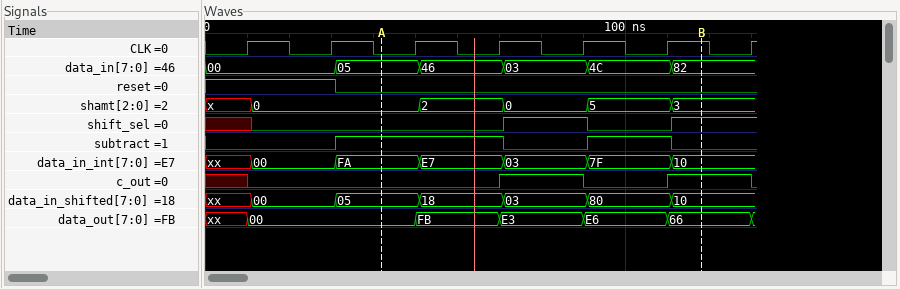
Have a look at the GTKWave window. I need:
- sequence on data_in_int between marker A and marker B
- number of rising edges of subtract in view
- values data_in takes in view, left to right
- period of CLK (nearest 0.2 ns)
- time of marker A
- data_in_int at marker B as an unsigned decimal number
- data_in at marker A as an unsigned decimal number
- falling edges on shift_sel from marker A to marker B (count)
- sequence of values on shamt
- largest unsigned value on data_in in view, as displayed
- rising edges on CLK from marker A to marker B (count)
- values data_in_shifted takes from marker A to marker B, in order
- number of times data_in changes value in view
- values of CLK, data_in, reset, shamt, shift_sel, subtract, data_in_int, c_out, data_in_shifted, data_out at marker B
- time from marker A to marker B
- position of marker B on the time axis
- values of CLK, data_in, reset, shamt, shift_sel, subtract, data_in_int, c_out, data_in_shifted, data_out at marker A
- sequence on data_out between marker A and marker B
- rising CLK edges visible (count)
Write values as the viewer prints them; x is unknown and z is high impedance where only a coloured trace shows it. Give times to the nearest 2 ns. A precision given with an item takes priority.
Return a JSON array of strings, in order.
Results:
["FA, E7, 03, 7F, 10", "2", "00, 05, 46, 03, 4C, 82", "20 ns", "42 ns", "16", "5", "1", "x, 0, 2, 0, 5, 3", "82", "4", "05, 18, 03, 80, 10", "5", "CLK=1, data_in=82, reset=0, shamt=3, shift_sel=1, subtract=0, data_in_int=10, c_out=1, data_in_shifted=10, data_out=66", "76 ns", "118 ns", "CLK=0, data_in=05, reset=0, shamt=0, shift_sel=0, subtract=1, data_in_int=FA, c_out=0, data_in_shifted=05, data_out=00", "00, FB, E3, E6, 66", "7"]
